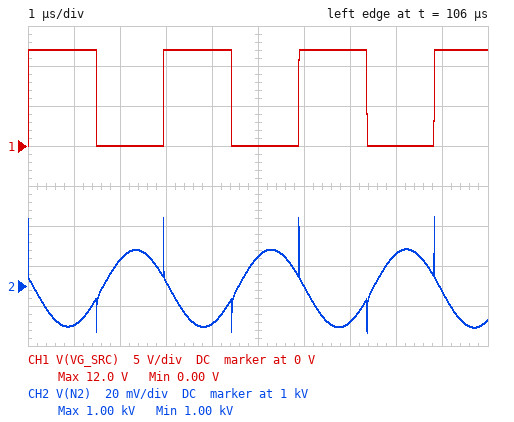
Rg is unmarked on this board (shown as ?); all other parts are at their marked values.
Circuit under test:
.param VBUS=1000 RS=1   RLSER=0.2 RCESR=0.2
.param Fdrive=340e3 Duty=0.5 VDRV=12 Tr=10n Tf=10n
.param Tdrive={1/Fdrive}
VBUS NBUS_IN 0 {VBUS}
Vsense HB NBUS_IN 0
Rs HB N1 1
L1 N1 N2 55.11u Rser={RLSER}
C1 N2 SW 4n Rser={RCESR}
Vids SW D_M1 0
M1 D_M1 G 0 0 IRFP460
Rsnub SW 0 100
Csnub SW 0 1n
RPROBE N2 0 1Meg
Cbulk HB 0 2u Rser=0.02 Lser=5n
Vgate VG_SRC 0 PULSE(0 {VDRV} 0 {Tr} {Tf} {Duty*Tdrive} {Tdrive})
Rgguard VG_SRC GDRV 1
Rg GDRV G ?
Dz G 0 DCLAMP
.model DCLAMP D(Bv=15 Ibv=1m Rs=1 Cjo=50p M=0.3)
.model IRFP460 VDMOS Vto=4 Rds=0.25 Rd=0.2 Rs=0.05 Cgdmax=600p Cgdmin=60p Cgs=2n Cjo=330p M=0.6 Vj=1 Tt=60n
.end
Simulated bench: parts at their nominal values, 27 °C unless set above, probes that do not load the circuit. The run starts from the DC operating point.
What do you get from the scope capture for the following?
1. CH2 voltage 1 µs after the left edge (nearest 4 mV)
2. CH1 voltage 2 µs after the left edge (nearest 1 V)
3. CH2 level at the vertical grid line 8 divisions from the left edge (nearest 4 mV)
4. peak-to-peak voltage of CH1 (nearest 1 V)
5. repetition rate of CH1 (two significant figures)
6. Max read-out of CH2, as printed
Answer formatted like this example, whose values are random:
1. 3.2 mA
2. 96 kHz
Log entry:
1. 999.980 V
2. 0 V
3. 1.000016 kV
4. 12 V
5. 340 kHz
6. 1.00 kV
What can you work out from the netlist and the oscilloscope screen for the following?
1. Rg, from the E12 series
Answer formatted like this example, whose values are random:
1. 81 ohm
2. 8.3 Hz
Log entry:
1. 8.2 Ω
